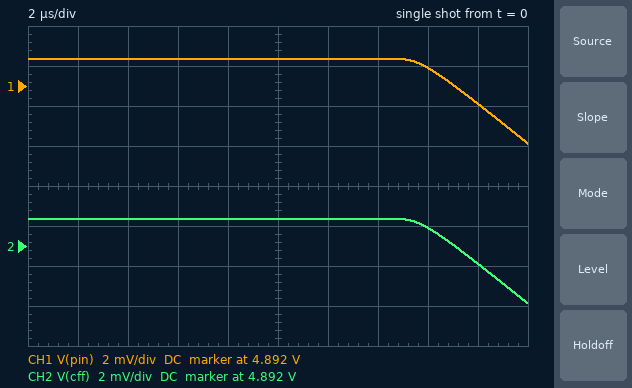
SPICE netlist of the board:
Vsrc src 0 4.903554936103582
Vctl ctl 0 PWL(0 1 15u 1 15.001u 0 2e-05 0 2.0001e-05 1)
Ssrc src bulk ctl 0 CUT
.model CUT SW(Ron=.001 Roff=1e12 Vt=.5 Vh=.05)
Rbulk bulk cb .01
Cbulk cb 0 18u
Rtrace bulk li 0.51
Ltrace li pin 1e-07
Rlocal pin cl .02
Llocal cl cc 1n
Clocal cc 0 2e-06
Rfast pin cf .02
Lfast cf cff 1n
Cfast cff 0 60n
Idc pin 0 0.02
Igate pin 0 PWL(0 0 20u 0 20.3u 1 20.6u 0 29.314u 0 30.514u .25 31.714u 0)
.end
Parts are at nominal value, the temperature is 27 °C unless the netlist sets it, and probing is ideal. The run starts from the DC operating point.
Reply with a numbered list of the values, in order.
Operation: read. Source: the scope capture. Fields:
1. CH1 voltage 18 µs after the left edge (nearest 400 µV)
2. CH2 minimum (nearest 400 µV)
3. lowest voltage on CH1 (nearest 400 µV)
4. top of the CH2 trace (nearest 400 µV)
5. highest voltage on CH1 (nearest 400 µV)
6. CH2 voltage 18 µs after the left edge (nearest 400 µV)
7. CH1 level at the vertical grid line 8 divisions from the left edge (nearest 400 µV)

1. 4.8912 V
2. 4.8892 V
3. 4.8892 V
4. 4.8932 V
5. 4.8932 V
6. 4.8912 V
7. 4.8928 V
